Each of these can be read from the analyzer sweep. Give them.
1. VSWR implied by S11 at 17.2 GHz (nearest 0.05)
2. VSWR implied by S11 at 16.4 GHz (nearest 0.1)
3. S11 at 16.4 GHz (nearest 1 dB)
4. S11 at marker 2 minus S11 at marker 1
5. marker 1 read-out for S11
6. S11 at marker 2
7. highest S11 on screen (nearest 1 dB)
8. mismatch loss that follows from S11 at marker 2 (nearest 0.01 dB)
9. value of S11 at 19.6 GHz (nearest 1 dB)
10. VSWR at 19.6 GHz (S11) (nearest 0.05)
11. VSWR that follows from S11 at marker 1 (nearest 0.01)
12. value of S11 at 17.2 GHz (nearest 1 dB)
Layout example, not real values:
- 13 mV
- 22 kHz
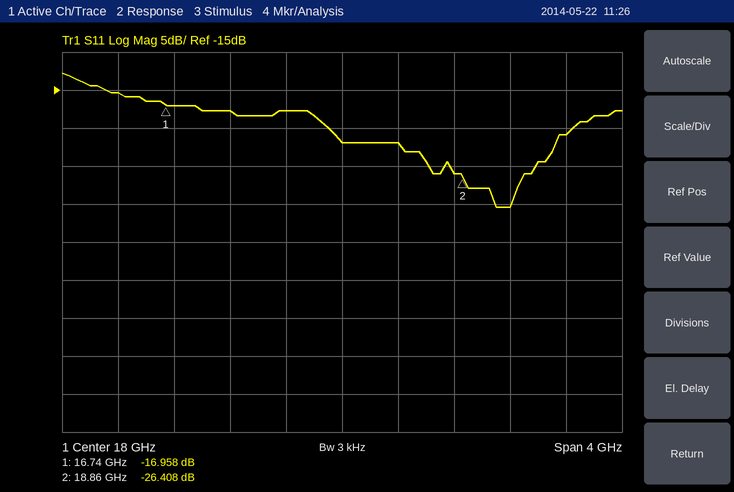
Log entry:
- 1.30
- 1.4
- -15 dB
- -9.450 dB
- -16.958 dB
- -26.408 dB
- -13 dB
- 0.01 dB
- -21 dB
- 1.20
- 1.33
- -18 dB
